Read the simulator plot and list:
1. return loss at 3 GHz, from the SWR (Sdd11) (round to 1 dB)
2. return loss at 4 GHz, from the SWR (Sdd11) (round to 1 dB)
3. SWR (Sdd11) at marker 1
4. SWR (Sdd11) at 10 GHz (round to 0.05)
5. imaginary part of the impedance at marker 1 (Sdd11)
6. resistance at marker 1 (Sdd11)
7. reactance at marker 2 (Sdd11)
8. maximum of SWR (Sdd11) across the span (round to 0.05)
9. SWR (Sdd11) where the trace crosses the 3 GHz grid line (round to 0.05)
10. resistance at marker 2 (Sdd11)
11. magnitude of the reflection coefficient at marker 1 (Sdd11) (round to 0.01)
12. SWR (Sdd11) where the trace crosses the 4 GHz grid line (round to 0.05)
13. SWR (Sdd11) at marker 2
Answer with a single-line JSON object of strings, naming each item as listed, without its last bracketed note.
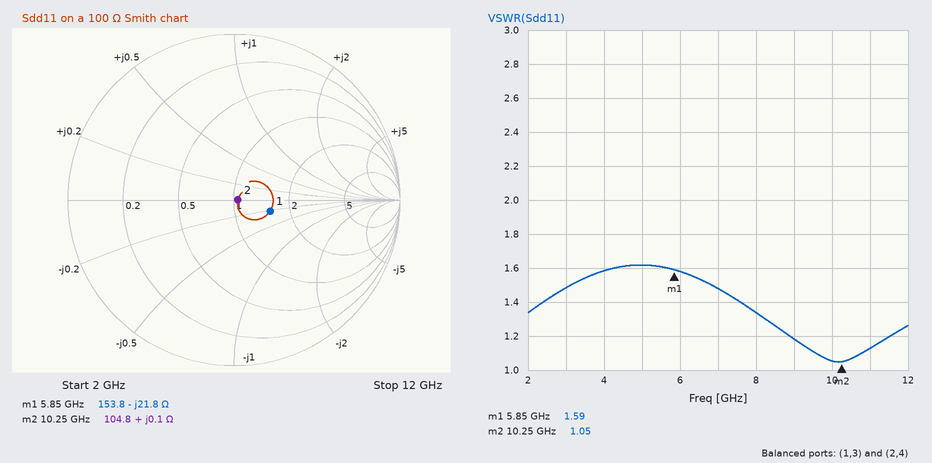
{"return loss at 3 GHz, from the SWR (Sdd11)": "14 dB", "return loss at 4 GHz, from the SWR (Sdd11)": "13 dB", "SWR (Sdd11) at marker 1": "1.59", "SWR (Sdd11) at 10 GHz": "1.05", "imaginary part of the impedance at marker 1": "-21.8 Ω", "resistance at marker 1": "153.8 Ω", "reactance at marker 2": "+0.1 Ω", "maximum of SWR (Sdd11) across the span": "1.60", "SWR (Sdd11) where the trace crosses the 3 GHz grid line": "1.50", "resistance at marker 2": "104.8 Ω", "magnitude of the reflection coefficient at marker 1 (Sdd11)": "0.23", "SWR (Sdd11) where the trace crosses the 4 GHz grid line": "1.60", "SWR (Sdd11) at marker 2": "1.05"}
